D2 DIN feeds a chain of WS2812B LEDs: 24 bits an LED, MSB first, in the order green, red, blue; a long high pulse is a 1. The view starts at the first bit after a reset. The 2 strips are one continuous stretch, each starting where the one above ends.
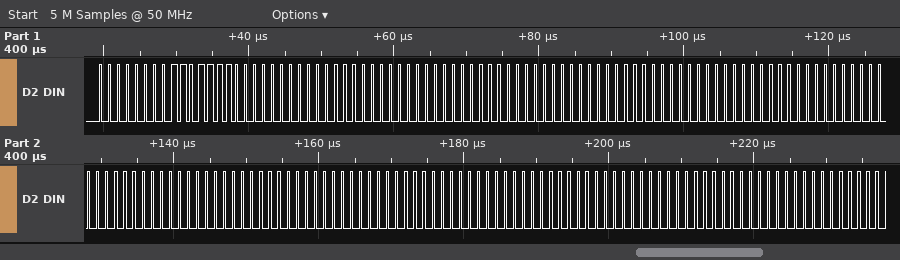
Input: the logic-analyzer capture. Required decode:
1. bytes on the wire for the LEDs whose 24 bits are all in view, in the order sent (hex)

00 DE 00 00 00 00 00 00 00 00 00 00 00 00 00 00 00 00 00 00 00
